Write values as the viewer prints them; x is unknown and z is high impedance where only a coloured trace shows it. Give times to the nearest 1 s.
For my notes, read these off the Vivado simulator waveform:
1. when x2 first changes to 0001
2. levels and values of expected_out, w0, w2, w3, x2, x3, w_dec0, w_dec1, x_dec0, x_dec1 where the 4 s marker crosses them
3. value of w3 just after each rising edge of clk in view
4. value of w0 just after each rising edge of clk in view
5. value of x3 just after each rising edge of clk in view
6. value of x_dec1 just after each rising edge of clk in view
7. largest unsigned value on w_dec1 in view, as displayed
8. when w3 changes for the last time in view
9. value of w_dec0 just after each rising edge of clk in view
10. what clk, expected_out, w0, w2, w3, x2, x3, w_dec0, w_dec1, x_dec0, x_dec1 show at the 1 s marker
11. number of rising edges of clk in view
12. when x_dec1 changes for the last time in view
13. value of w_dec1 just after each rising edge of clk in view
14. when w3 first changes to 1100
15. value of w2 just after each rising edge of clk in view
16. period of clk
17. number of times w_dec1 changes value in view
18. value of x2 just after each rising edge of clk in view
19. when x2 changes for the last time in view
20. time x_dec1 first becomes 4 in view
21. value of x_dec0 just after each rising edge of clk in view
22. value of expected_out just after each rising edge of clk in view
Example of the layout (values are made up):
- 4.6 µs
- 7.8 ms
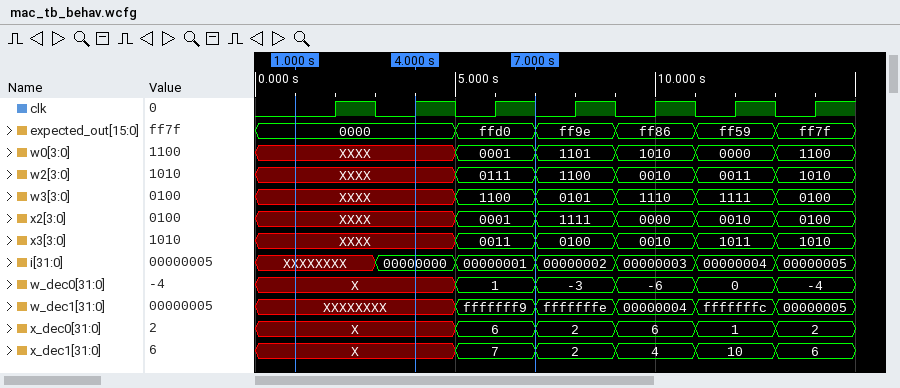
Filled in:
- 5 s
- expected_out=0000, w0=XXXX, w2=XXXX, w3=XXXX, x2=XXXX, x3=XXXX, w_dec0=X, w_dec1=XXXXXXXX, x_dec0=X, x_dec1=X
- XXXX, XXXX, 1100, 0101, 1110, 1111, 0100
- XXXX, XXXX, 0001, 1101, 1010, 0000, 1100
- XXXX, XXXX, 0011, 0100, 0010, 1011, 1010
- X, X, 7, 2, 4, 10, 6
- fffffffe
- 13 s
- X, X, 1, -3, -6, 0, -4
- clk=0, expected_out=0000, w0=XXXX, w2=XXXX, w3=XXXX, x2=XXXX, x3=XXXX, w_dec0=X, w_dec1=XXXXXXXX, x_dec0=X, x_dec1=X
- 7
- 13 s
- XXXXXXXX, XXXXXXXX, fffffff9, fffffffe, 00000004, fffffffc, 00000005
- 5 s
- XXXX, XXXX, 0111, 1100, 0010, 0011, 1010
- 2 s
- 5
- XXXX, XXXX, 0001, 1111, 0000, 0010, 0100
- 13 s
- 9 s
- X, X, 6, 2, 6, 1, 2
- 0000, 0000, ffd0, ff9e, ff86, ff59, ff7f
